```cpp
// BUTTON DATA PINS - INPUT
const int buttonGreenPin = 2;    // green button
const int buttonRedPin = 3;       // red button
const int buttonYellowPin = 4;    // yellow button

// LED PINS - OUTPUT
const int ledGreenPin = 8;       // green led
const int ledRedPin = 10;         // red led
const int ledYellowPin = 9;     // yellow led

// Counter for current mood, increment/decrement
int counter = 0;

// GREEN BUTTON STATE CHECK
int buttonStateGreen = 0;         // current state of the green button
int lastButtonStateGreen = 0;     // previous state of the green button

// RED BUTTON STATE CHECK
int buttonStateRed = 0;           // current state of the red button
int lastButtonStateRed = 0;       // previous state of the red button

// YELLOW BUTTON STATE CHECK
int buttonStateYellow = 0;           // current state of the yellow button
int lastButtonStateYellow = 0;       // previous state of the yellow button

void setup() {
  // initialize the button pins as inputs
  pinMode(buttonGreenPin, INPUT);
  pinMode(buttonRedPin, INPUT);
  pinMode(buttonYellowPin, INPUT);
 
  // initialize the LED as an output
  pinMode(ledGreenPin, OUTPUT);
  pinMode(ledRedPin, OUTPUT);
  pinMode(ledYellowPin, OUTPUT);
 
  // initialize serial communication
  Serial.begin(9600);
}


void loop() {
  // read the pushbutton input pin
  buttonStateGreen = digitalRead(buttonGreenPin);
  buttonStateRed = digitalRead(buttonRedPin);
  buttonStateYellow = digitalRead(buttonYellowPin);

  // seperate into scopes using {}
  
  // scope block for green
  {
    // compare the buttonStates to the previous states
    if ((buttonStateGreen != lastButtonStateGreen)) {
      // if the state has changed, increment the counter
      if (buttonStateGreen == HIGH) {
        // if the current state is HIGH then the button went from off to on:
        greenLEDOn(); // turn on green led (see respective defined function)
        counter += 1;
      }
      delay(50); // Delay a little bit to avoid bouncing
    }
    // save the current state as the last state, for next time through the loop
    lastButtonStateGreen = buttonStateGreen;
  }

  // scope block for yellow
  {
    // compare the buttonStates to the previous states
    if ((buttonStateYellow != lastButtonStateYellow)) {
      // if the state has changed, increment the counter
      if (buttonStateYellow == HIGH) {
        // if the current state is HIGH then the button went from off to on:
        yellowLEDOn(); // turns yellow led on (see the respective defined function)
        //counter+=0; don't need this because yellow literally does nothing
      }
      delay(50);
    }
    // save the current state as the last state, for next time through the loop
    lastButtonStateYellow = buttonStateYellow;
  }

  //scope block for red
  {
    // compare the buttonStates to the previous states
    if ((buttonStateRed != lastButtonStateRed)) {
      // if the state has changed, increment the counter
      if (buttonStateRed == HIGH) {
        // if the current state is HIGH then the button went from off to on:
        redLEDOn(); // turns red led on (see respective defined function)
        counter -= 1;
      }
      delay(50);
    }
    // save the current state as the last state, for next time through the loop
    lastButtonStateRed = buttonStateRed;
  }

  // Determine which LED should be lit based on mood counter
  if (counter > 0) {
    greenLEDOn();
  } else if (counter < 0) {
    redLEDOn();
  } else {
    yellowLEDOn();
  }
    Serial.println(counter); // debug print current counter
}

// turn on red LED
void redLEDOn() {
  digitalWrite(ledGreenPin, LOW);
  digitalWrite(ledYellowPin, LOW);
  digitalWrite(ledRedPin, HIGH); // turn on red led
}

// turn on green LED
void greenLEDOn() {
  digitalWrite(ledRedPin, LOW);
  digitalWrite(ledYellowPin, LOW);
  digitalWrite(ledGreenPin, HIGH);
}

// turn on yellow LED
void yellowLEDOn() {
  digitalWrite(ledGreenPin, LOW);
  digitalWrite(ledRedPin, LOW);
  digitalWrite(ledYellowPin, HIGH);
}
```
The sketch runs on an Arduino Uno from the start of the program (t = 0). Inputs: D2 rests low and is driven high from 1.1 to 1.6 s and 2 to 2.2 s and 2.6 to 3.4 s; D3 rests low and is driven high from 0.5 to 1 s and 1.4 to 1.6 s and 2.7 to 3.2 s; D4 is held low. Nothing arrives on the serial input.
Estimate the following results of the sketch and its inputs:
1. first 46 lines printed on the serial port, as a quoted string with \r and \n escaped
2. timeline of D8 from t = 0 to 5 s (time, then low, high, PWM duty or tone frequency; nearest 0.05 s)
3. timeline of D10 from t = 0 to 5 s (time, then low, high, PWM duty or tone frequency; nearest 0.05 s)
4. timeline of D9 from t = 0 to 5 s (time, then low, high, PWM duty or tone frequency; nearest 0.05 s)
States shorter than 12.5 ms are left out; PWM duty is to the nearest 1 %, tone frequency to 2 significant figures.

"0\r\n0\r\n0\r\n0\r\n0\r\n0\r\n0\r\n0\r\n0\r\n0\r\n0\r\n0\r\n0\r\n0\r\n0\r\n0\r\n0\r\n0\r\n0\r\n0\r\n0\r\n0\r\n0\r\n0\r\n0\r\n0\r\n0\r\n0\r\n0\r\n0\r\n0\r\n0\r\n0\r\n0\r\n0\r\n0\r\n0\r\n0\r\n0\r\n0\r\n0\r\n0\r\n0\r\n0\r\n0\r\n0\r\n"
0 s low; 1.1 s high; 1.15 s low; 2 s high; 2.05 s low; 2.6 s high; 2.7 s low
0 s low; 0.5 s high; 1.1 s low; 1.4 s high; 2 s low; 2.7 s high; 2.75 s low
0 s high; 0.5 s low; 1.15 s high; 1.4 s low; 2.05 s high; 2.6 s low; 2.75 s high
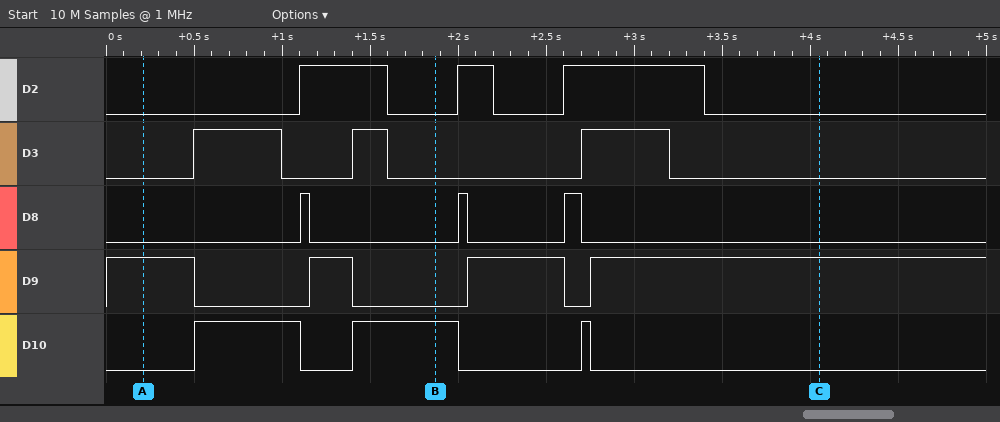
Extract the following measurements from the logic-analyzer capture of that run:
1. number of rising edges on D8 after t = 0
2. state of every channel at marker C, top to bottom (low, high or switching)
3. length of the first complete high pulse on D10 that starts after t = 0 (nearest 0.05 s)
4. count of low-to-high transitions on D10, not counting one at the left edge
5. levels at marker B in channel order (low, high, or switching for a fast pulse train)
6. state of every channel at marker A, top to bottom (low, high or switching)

3
D2 low, D3 low, D8 low, D9 high, D10 low
0.60 s
3
D2 low, D3 low, D8 low, D9 low, D10 high
D2 low, D3 low, D8 low, D9 high, D10 low
